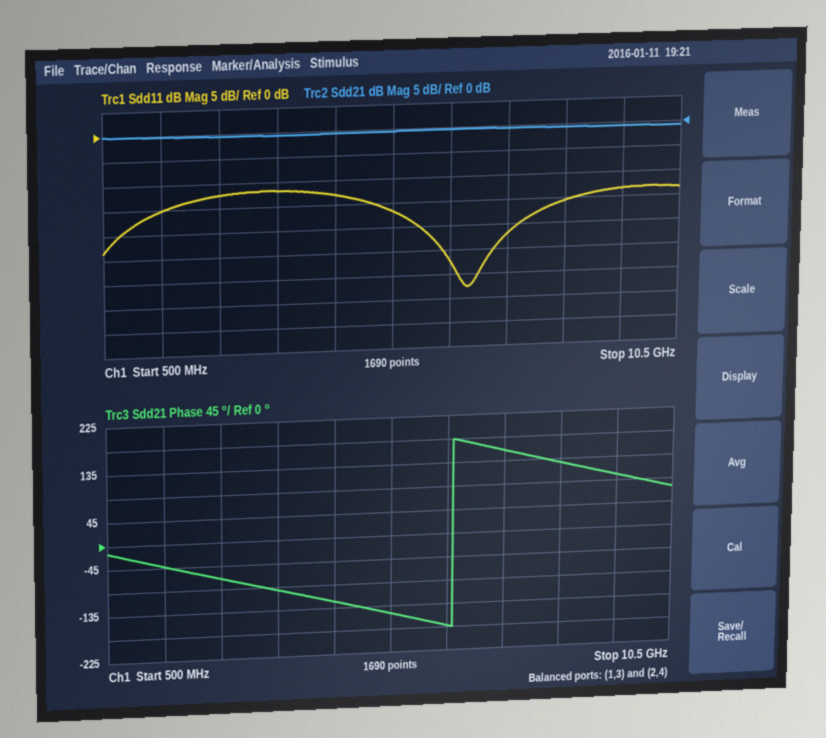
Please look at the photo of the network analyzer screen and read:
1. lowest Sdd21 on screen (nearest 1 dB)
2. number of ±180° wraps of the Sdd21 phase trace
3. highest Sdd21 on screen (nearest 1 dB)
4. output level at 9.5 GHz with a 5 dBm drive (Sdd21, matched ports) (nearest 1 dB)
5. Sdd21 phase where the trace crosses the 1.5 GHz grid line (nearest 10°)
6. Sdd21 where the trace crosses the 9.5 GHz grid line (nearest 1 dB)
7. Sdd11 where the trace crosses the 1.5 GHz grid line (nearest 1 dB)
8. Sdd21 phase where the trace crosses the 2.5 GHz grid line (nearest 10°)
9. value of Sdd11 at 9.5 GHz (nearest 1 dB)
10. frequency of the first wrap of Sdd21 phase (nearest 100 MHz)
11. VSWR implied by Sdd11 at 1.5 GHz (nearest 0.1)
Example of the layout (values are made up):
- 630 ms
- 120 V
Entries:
- -1 dB
- 1
- 0 dB
- 4 dBm
- -40°
- -1 dB
- -15 dB
- -70°
- -13 dB
- 6.6 GHz
- 1.4
